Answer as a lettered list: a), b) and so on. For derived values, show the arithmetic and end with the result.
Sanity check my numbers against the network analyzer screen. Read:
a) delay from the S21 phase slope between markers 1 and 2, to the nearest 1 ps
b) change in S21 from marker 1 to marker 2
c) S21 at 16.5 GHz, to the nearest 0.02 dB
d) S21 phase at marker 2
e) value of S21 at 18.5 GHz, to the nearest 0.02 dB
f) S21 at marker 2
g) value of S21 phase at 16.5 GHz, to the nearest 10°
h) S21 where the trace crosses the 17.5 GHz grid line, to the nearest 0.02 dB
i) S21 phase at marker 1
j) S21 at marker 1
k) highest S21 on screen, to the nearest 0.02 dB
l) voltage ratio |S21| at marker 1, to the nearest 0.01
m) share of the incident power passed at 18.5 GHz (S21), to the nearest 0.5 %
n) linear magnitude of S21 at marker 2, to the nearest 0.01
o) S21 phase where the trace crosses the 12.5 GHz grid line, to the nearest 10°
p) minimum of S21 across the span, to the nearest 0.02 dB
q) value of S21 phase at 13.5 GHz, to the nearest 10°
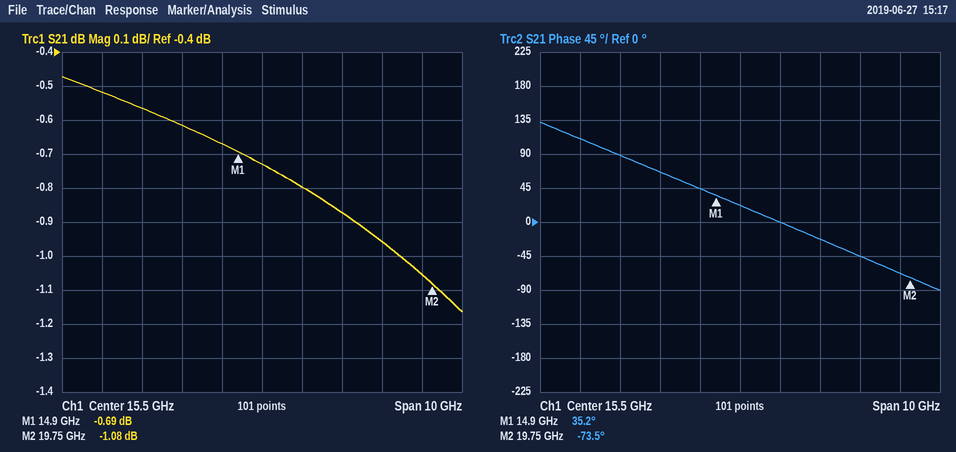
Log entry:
a) −(-73.5° − (35.2°))/(360° × 4.85 GHz) ≈ 62 ps
b) -1.08 − (-0.69) = -0.39 dB
c) -0.80 dB
d) -73.5°
e) -0.96 dB
f) -1.08 dB
g) 0°
h) -0.88 dB
i) 35.2°
j) -0.69 dB
k) -0.48 dB
l) 10^(-0.69/20) ≈ 0.92
m) 10^(-0.96/10) ≈ 80.2 %, so 80.0 % to the nearest 0.5 %
n) 10^(-1.08/20) ≈ 0.88
o) 90°
p) -1.16 dB
q) 70°
